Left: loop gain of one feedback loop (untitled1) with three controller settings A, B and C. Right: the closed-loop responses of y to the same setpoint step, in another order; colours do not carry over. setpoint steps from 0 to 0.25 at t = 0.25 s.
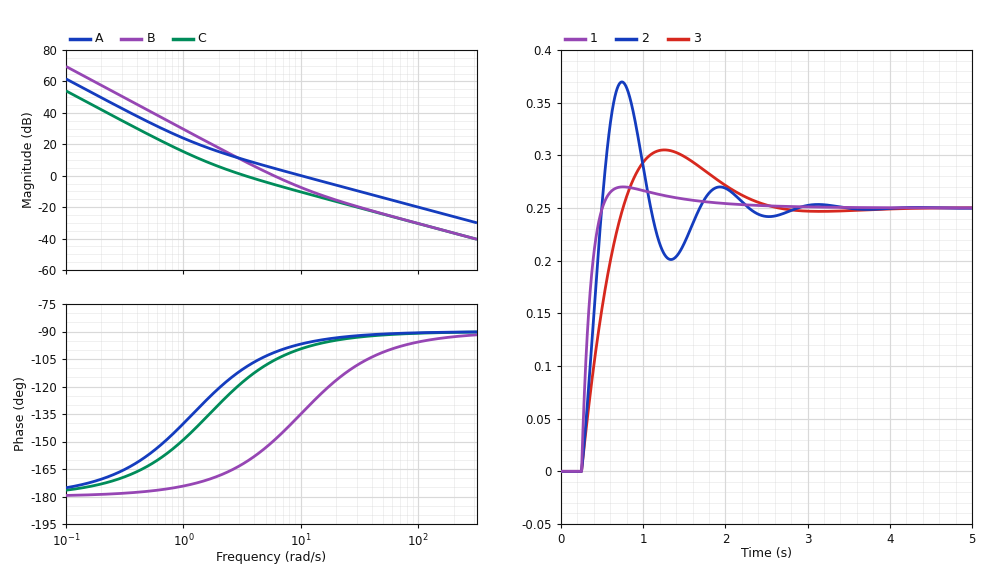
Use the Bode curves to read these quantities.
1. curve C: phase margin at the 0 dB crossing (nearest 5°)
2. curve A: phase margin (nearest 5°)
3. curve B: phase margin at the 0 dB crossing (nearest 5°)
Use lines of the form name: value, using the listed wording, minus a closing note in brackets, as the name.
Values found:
curve C: phase margin at the 0 dB crossing: 65°
curve A: phase margin: 85°
curve B: phase margin at the 0 dB crossing: 30°
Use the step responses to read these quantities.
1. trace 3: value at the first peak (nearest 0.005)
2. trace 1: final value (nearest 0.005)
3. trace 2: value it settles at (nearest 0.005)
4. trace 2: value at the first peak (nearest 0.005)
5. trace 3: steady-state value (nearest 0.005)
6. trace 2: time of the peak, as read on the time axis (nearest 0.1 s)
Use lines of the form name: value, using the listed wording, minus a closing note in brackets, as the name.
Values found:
trace 3: value at the first peak: 0.305
trace 1: final value: 0.250
trace 2: value it settles at: 0.250
trace 2: value at the first peak: 0.370
trace 3: steady-state value: 0.250
trace 2: time of the peak, as read on the time axis: 0.7 s
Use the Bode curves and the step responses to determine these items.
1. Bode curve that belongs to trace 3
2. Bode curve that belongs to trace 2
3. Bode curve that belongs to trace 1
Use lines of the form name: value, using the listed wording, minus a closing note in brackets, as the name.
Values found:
Bode curve that belongs to trace 3: C
Bode curve that belongs to trace 2: B
Bode curve that belongs to trace 1: A
